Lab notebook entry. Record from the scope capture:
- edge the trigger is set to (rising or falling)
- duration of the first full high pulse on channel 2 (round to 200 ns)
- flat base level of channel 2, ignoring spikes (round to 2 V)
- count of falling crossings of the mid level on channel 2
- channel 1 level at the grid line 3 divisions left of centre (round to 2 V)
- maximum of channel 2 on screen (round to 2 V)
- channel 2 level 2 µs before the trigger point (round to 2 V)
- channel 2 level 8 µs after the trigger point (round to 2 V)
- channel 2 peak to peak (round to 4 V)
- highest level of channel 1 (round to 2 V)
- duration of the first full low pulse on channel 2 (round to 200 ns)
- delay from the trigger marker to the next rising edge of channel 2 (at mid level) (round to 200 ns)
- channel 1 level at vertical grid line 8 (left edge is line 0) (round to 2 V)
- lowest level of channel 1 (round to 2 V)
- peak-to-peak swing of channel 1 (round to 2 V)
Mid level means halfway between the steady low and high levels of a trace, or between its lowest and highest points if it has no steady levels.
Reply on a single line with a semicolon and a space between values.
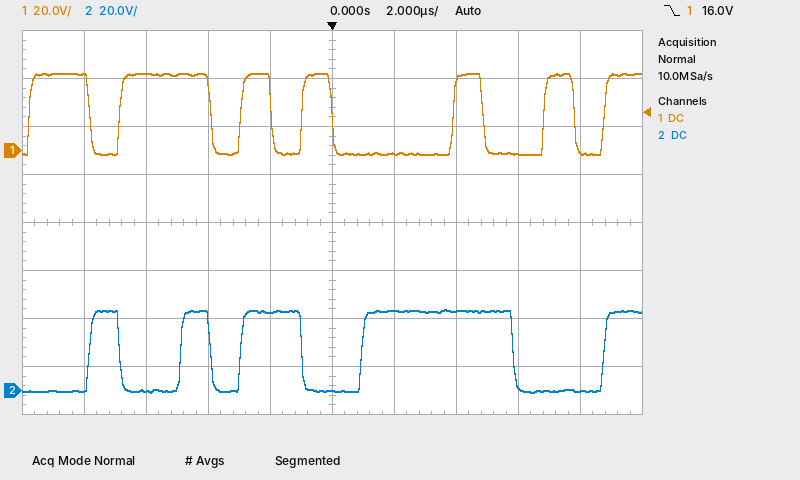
falling; 1.0 µs; 0 V; 4; 32 V; 34 V; 32 V; 0 V; 36 V; 32 V; 2.0 µs; 1.0 µs; -2 V; -2 V; 34 V
